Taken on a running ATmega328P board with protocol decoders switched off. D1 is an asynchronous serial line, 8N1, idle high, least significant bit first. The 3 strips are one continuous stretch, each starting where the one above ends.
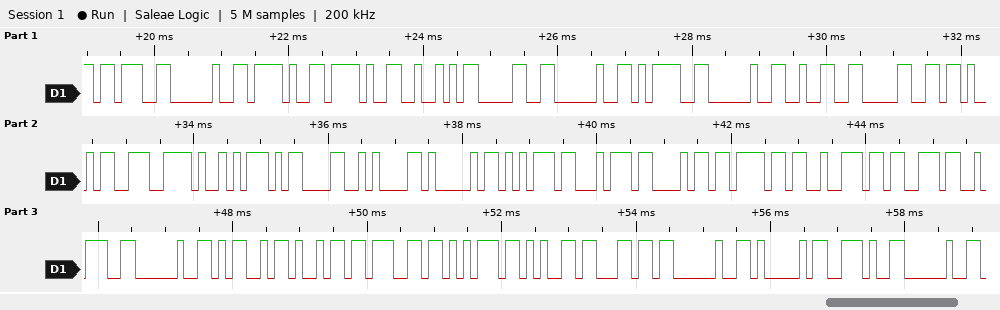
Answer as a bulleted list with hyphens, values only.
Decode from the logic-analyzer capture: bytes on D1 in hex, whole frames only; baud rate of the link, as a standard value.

- 3B 20 2F 2F 52 30 20 3D 20 32 30 4B CE A9 0D 0A 41 75 74 68 6F 72 73 3A 20 4D 69 67 75 65 6C 20 41 2E 20
- 9600 baud
